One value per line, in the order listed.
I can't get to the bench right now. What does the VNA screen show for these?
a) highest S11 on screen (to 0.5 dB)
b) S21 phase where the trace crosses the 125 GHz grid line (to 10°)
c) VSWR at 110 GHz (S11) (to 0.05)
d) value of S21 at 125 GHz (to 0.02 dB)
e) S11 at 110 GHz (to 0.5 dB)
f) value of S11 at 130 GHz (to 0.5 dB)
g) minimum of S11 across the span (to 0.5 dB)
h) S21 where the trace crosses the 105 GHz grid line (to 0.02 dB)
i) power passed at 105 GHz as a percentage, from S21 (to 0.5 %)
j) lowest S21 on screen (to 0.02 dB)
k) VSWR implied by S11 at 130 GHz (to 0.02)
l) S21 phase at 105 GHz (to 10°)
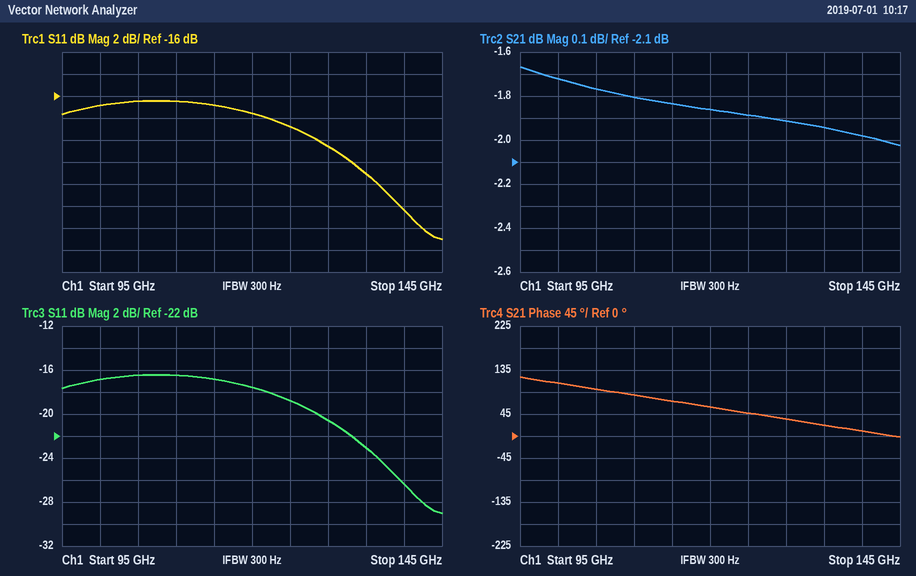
-16.5 dB
50°
1.35
-1.88 dB
-16.5 dB
-20.5 dB
-29.0 dB
-1.76 dB
66.5 %
-2.02 dB
1.20
100°
